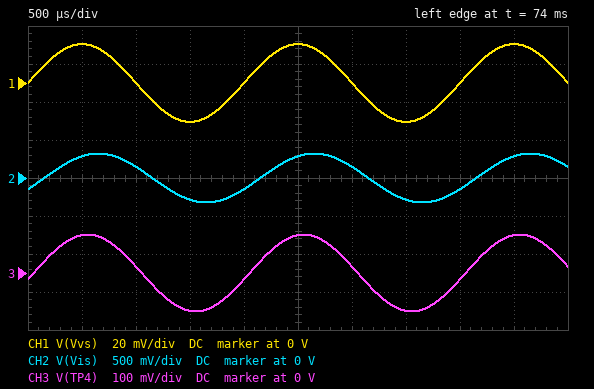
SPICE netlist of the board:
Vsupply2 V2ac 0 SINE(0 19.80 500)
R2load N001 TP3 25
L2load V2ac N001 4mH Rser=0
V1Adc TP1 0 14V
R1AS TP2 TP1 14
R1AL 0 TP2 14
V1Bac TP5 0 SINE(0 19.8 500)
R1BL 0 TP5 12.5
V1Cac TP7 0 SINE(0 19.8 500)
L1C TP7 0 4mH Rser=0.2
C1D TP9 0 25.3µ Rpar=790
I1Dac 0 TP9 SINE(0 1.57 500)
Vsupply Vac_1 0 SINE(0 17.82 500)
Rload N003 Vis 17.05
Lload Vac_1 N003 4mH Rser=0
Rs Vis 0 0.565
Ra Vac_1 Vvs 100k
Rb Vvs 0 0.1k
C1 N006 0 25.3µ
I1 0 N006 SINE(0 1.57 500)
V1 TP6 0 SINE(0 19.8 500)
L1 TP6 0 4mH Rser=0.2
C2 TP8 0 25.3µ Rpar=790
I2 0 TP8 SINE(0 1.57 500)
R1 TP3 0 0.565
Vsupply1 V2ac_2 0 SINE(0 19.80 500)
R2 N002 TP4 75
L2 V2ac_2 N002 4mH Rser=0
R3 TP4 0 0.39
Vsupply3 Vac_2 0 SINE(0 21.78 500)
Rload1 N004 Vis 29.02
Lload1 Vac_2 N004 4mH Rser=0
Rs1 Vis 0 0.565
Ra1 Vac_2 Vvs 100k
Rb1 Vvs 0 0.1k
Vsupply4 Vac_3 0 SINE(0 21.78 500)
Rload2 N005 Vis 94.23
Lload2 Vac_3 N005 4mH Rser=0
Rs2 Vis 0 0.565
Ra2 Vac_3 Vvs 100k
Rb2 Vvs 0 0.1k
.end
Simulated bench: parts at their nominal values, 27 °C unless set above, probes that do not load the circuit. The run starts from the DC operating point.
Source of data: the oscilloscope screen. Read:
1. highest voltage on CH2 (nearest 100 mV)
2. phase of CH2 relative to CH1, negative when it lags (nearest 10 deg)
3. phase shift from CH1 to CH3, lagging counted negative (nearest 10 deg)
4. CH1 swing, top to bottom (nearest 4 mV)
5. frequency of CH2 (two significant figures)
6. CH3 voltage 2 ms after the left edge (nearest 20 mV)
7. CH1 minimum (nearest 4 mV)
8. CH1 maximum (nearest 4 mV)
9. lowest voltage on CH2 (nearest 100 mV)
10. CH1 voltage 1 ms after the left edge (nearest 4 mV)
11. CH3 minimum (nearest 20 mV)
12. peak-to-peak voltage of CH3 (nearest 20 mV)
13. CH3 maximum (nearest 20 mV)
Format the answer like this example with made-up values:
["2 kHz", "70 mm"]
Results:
["300 mV", "-30 deg", "-10 deg", "40 mV", "500 Hz", "-20 mV", "-20 mV", "20 mV", "-300 mV", "0 V", "-100 mV", "200 mV", "100 mV"]
